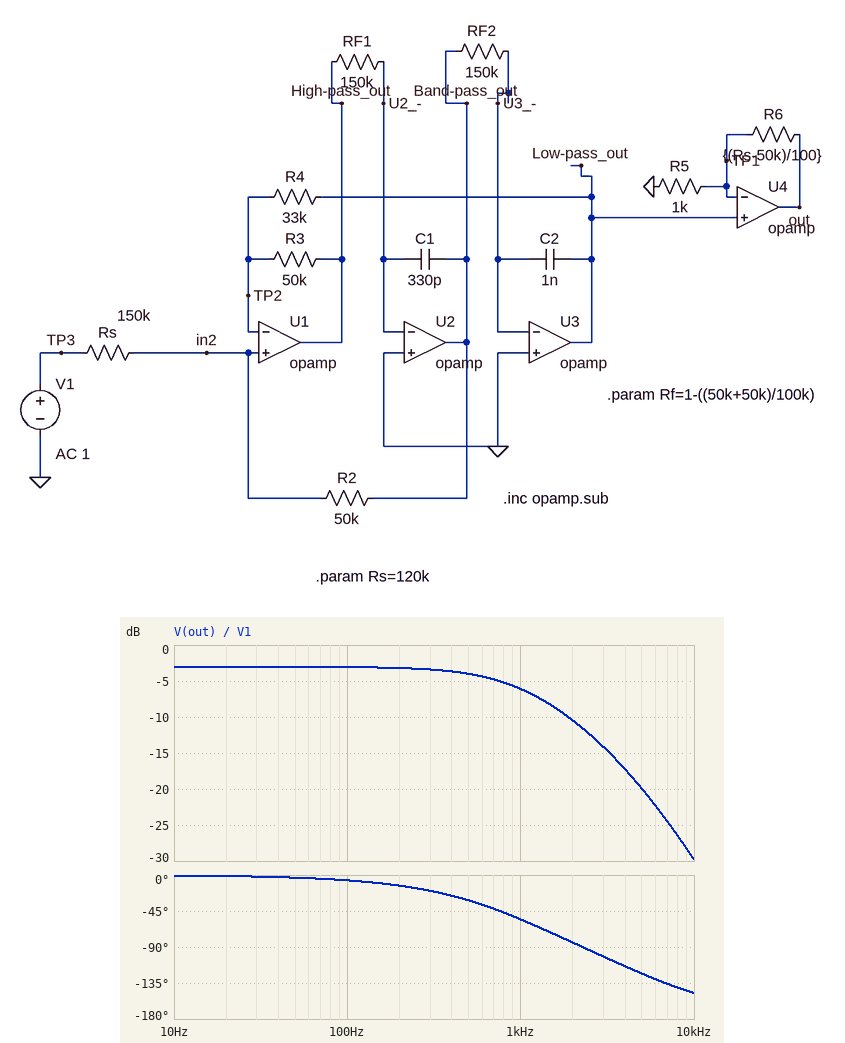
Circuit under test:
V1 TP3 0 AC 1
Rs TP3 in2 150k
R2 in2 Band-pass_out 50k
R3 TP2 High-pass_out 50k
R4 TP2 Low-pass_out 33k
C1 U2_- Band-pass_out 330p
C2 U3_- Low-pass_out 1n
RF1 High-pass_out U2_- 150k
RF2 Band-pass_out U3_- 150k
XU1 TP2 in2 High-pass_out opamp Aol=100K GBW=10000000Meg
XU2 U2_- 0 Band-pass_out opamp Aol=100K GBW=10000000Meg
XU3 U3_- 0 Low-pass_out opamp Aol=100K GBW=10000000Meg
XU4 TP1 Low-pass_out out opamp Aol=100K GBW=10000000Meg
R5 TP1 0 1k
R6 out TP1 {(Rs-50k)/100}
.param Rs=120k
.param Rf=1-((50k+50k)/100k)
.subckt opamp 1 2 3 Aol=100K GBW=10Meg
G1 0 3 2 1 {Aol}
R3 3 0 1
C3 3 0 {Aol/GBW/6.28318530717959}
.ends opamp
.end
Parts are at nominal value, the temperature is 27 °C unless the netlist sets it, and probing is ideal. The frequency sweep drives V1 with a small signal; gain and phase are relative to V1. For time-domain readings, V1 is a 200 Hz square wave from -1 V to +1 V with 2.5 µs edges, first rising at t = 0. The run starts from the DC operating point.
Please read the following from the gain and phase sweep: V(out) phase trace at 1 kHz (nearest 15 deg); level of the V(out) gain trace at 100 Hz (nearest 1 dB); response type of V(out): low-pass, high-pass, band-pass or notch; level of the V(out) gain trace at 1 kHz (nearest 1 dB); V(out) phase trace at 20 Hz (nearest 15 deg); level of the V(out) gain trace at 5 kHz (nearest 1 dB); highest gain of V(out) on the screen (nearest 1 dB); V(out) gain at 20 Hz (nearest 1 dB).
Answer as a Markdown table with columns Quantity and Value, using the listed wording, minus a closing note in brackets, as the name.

| Quantity | Value |
|---|---|
| V(out) phase trace at 1 kHz | -60 deg |
| level of the V(out) gain trace at 100 Hz | -3 dB |
| response type of V(out): low-pass, high-pass, band-pass or notch | low-pass |
| level of the V(out) gain trace at 1 kHz | -6 dB |
| V(out) phase trace at 20 Hz | 0 deg |
| level of the V(out) gain trace at 5 kHz | -20 dB |
| highest gain of V(out) on the screen | -3 dB |
| V(out) gain at 20 Hz | -3 dB |
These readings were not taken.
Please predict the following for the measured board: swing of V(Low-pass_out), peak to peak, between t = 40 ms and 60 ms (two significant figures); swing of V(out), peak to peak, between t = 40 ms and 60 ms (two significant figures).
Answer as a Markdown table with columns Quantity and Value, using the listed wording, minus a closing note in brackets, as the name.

| Quantity | Value |
|---|---|
| swing of V(Low-pass_out), peak to peak, between t = 40 ms and 60 ms | 830 mV |
| swing of V(out), peak to peak, between t = 40 ms and 60 ms | 1.4 V |
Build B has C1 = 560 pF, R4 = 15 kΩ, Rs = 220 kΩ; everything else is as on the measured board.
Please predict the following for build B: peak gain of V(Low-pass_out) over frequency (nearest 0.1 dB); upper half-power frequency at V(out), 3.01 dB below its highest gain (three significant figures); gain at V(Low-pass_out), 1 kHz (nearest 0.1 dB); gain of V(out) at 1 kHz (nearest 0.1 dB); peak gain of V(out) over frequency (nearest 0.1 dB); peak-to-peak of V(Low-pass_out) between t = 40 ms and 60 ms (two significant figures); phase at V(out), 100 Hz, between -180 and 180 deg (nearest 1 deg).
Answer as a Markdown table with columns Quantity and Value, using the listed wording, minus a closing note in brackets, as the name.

| Quantity | Value |
|---|---|
| peak gain of V(Low-pass_out) over frequency | -12.4 dB |
| upper half-power frequency at V(out), 3.01 dB below its highest gain | 1.17 kHz |
| gain at V(Low-pass_out), 1 kHz | -14.7 dB |
| gain of V(out) at 1 kHz | -10.1 dB |
| peak gain of V(out) over frequency | -7.8 dB |
| peak-to-peak of V(Low-pass_out) between t = 40 ms and 60 ms | 480 mV |
| phase at V(out), 100 Hz, between -180 and 180 deg | -6 deg |
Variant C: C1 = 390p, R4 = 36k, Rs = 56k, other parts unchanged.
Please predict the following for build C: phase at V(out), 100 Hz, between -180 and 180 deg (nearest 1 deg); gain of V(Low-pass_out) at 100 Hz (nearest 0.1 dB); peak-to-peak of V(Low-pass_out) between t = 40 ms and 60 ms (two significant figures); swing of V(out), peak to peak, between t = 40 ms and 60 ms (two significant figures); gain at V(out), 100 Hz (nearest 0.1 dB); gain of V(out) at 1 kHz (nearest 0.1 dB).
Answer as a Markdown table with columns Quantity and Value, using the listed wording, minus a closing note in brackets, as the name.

| Quantity | Value |
|---|---|
| phase at V(out), 100 Hz, between -180 and 180 deg | -5 deg |
| gain of V(Low-pass_out) at 100 Hz | -1.8 dB |
| peak-to-peak of V(Low-pass_out) between t = 40 ms and 60 ms | 1.6 V |
| swing of V(out), peak to peak, between t = 40 ms and 60 ms | 2.8 V |
| gain at V(out), 100 Hz | 2.8 dB |
| gain of V(out) at 1 kHz | 1.7 dB |
